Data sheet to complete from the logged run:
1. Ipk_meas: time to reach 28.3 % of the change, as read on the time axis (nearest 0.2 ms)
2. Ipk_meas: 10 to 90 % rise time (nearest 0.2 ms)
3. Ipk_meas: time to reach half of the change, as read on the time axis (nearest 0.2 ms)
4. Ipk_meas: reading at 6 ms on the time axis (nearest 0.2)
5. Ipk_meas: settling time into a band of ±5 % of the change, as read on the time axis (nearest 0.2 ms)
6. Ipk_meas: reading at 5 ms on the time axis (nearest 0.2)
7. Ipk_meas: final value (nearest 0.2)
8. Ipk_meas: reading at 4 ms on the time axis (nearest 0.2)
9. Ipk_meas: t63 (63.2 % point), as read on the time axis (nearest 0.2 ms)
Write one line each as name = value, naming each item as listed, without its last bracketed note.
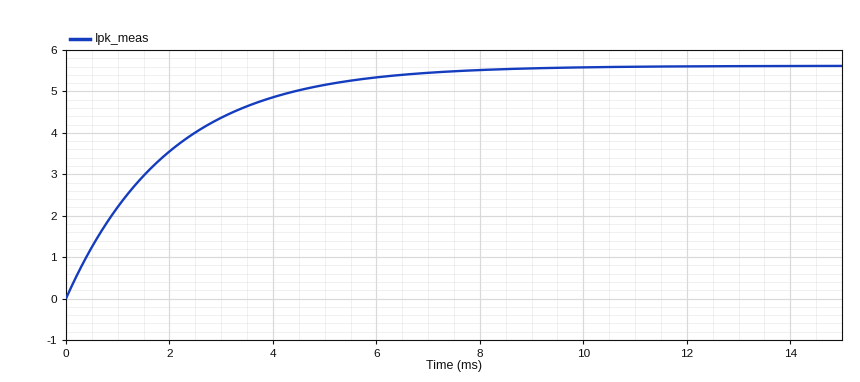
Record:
Ipk_meas: time to reach 28.3 % of the change, as read on the time axis = 0.6 ms
Ipk_meas: 10 to 90 % rise time = 4.4 ms
Ipk_meas: time to reach half of the change, as read on the time axis = 1.4 ms
Ipk_meas: reading at 6 ms on the time axis = 5.4
Ipk_meas: settling time into a band of ±5 % of the change, as read on the time axis = 6.0 ms
Ipk_meas: reading at 5 ms on the time axis = 5.2
Ipk_meas: final value = 5.6
Ipk_meas: reading at 4 ms on the time axis = 4.8
Ipk_meas: t63 (63.2 % point), as read on the time axis = 2.0 ms
